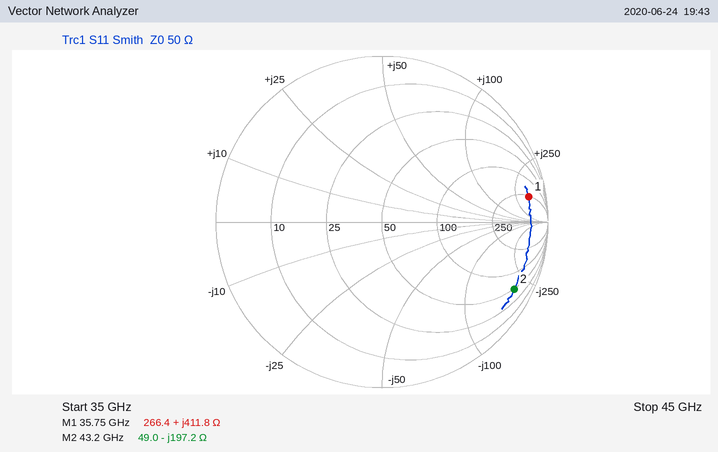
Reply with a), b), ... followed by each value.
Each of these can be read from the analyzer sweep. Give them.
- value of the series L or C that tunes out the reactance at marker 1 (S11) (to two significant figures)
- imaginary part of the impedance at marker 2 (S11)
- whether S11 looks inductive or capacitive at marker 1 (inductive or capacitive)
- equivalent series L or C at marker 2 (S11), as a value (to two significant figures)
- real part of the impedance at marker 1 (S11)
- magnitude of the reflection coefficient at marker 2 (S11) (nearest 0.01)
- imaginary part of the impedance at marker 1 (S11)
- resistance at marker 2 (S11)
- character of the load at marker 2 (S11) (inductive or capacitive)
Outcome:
a) 11 fF
b) -197.2 Ω
c) inductive
d) 19 fF
e) 266.4 Ω
f) 0.89
g) +411.8 Ω
h) 49.0 Ω
i) capacitive
